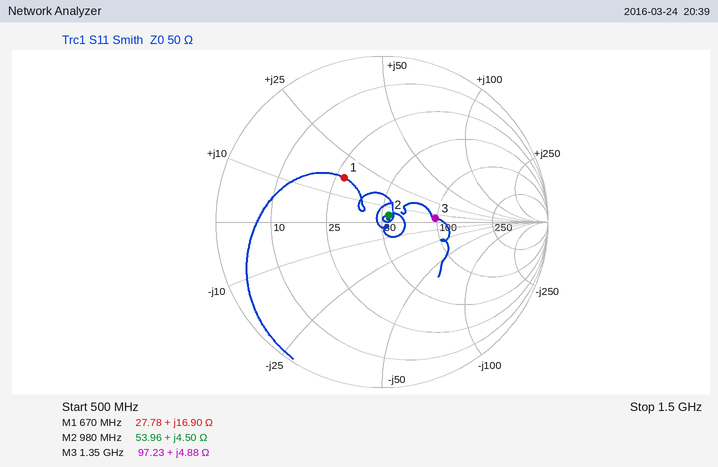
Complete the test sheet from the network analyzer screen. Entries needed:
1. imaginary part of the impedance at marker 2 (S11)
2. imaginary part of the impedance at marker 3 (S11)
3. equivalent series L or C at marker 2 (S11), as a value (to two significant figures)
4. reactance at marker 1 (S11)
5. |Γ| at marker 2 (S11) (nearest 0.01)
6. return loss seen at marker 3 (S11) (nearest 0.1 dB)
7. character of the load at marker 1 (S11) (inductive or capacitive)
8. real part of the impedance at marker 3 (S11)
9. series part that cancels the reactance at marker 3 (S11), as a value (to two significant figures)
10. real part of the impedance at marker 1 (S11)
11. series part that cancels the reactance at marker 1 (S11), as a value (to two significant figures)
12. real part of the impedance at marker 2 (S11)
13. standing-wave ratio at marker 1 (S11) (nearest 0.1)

+4.50 Ω
+4.88 Ω
730 pH
+16.90 Ω
0.06
9.8 dB
inductive
97.23 Ω
24 pF
27.78 Ω
14 pF
53.96 Ω
2.1
